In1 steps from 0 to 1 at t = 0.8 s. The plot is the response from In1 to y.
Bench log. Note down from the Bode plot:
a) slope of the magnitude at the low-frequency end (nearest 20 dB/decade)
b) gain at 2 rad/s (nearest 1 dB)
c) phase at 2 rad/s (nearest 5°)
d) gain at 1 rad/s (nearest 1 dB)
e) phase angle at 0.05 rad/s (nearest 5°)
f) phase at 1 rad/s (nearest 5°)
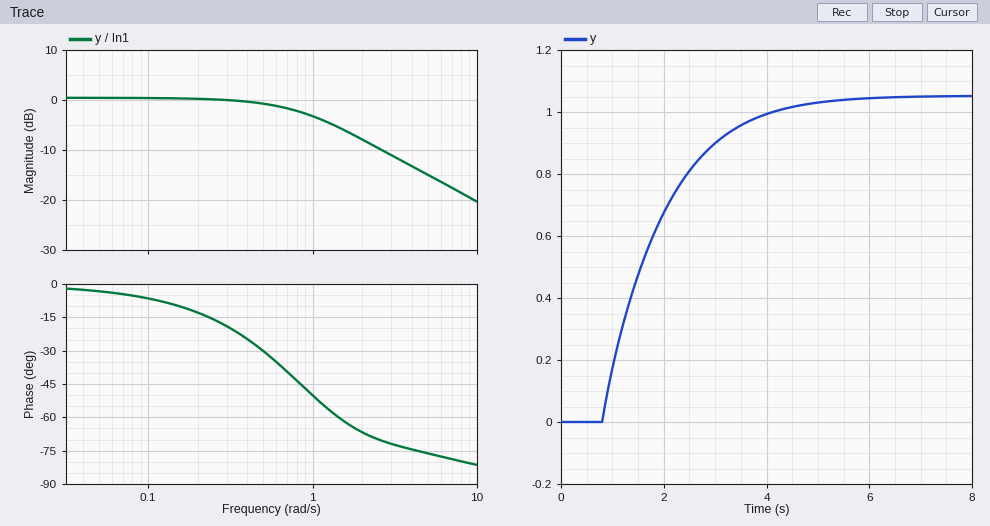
0 dB/decade
-8 dB
-65°
-3 dB
-5°
-50°
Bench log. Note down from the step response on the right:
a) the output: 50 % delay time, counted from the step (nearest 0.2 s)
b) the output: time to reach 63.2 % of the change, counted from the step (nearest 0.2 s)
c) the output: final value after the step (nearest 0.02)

0.8 s
1.2 s
1.06
